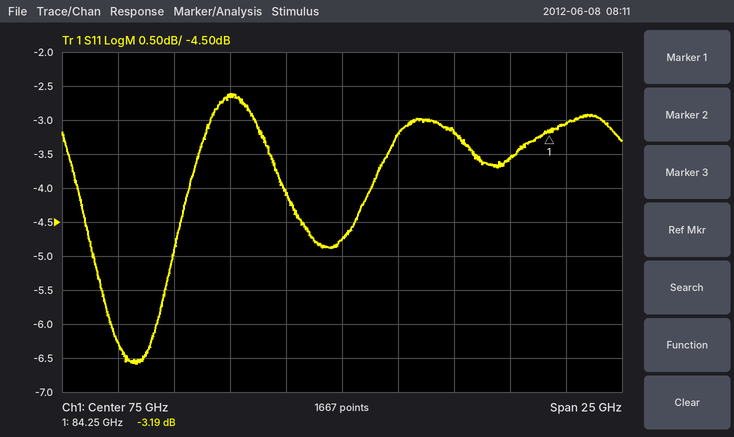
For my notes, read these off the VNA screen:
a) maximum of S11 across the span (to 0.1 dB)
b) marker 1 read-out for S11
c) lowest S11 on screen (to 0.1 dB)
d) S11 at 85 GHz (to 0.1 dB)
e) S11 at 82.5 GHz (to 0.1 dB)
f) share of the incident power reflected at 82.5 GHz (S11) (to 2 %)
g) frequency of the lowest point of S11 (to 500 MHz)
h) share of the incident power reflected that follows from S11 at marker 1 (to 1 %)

-2.6 dB
-3.19 dB
-6.6 dB
-3.1 dB
-3.6 dB
44 %
66.0 GHz
48 %
